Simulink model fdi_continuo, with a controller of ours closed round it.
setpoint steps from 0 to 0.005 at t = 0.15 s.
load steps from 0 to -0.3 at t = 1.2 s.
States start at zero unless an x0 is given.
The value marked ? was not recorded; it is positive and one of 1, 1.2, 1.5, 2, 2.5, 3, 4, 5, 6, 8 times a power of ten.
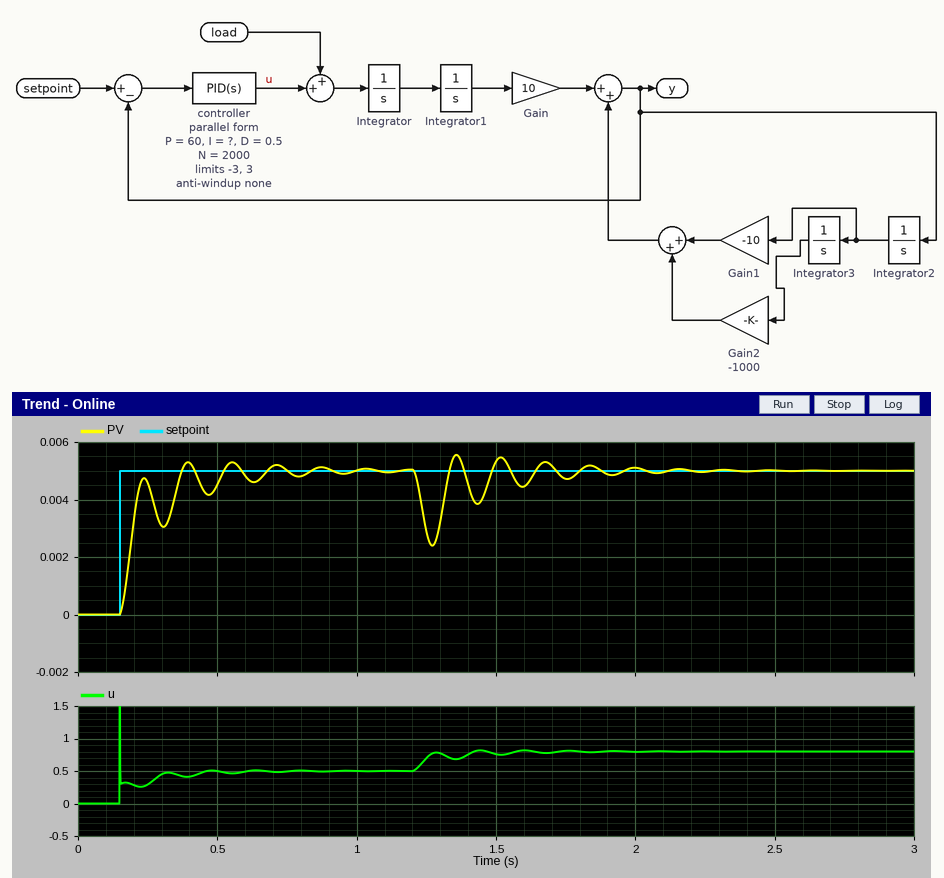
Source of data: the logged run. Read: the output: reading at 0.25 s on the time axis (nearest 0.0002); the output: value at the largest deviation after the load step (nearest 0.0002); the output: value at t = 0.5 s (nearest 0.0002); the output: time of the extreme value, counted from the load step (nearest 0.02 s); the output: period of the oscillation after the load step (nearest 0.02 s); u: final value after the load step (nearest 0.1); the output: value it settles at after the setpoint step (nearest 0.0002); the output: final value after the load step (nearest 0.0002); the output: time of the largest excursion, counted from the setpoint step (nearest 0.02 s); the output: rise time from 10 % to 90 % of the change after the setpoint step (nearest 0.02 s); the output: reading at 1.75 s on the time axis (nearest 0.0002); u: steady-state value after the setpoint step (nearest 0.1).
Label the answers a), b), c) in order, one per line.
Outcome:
a) 0.0046
b) 0.0024
c) 0.0046
d) 0.08 s
e) 0.16 s
f) 0.8
g) 0.0050
h) 0.0050
i) 0.24 s
j) 0.06 s
k) 0.0048
l) 0.5
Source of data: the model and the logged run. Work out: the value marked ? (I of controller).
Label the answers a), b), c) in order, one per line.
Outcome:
a) 1200
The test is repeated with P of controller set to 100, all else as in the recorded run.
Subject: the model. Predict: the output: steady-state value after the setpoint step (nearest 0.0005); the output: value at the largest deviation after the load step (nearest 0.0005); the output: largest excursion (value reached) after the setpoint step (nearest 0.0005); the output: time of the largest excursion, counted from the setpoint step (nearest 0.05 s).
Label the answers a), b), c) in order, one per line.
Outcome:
a) 0.0050
b) 0.0030
c) 0.0055
d) 0.20 s
